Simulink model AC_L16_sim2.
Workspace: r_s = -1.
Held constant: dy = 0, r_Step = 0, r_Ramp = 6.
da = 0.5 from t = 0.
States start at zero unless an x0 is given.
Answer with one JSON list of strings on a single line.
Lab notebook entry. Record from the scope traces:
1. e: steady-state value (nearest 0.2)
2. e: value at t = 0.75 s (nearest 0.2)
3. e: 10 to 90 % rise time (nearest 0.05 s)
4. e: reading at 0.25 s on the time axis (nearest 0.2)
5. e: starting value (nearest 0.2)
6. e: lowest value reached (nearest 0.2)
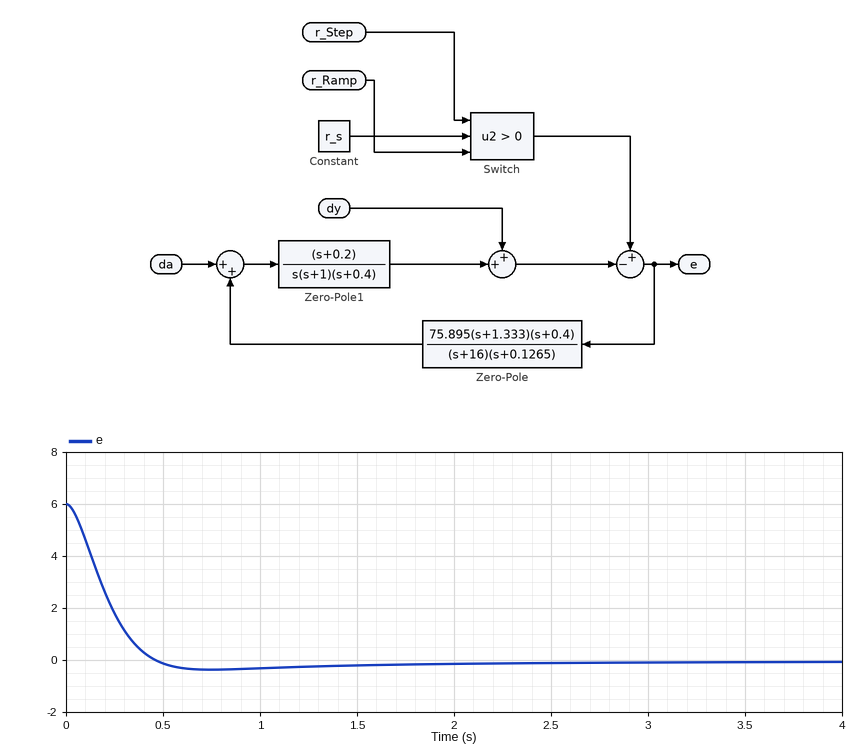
["0.0", "-0.4", "0.30 s", "1.8", "6.0", "-0.4"]
